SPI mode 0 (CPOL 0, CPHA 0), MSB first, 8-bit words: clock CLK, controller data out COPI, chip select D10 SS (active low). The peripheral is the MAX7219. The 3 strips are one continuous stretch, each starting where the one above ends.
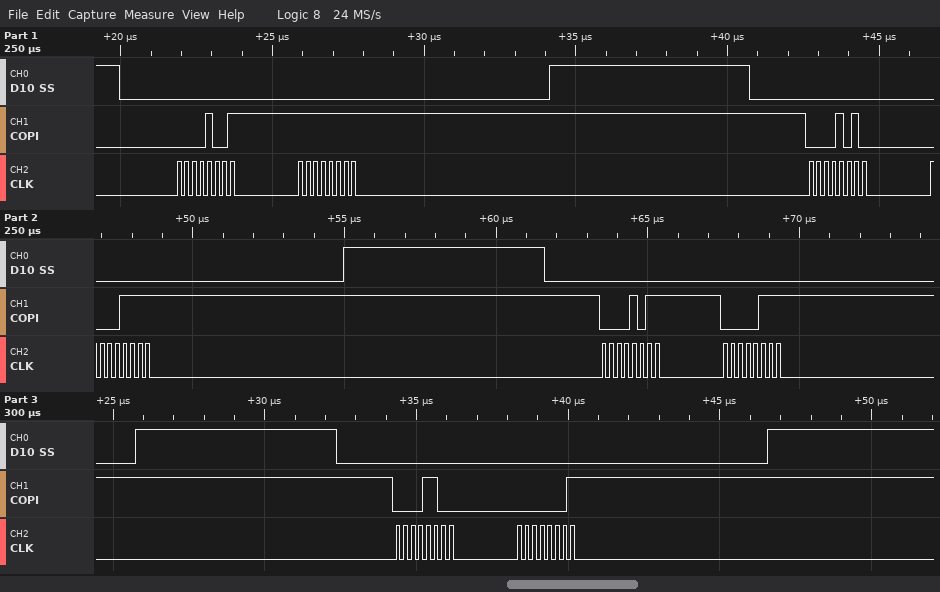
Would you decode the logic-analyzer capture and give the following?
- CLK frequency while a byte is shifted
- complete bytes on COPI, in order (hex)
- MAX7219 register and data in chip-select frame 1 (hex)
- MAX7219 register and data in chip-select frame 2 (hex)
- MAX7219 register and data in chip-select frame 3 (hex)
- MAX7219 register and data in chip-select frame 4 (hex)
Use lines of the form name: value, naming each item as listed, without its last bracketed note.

CLK frequency while a byte is shifted: 4 MHz
complete bytes on COPI, in order: 09 FF 0A 0F 0B 07 0C 01
MAX7219 register and data in chip-select frame 1: register 0x9, data 0xFF
MAX7219 register and data in chip-select frame 2: register 0xA, data 0x0F
MAX7219 register and data in chip-select frame 3: register 0xB, data 0x07
MAX7219 register and data in chip-select frame 4: register 0xC, data 0x01
